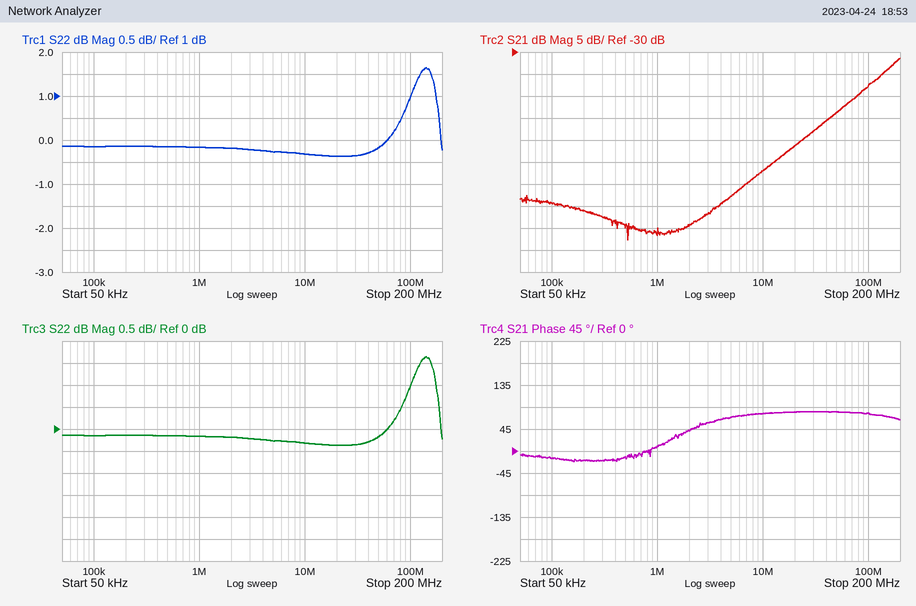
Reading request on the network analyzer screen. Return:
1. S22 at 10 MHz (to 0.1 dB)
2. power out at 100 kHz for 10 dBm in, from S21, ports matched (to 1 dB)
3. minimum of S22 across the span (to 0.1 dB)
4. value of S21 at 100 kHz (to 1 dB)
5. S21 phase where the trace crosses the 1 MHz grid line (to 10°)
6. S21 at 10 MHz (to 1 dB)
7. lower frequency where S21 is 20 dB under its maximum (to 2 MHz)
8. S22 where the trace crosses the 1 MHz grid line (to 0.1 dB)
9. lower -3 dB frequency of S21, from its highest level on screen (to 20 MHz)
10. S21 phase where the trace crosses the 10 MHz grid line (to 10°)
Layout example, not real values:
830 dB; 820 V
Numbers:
-0.3 dB; -54 dBm; -0.4 dB; -64 dB; 10°; -57 dB; 20 MHz; -0.2 dB; 140 MHz; 80°
